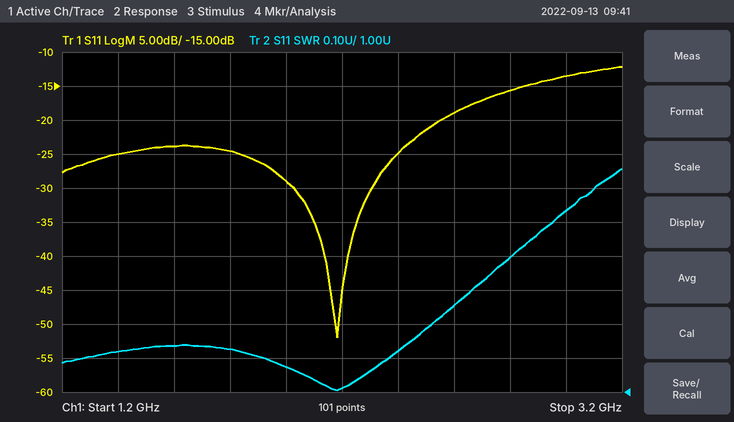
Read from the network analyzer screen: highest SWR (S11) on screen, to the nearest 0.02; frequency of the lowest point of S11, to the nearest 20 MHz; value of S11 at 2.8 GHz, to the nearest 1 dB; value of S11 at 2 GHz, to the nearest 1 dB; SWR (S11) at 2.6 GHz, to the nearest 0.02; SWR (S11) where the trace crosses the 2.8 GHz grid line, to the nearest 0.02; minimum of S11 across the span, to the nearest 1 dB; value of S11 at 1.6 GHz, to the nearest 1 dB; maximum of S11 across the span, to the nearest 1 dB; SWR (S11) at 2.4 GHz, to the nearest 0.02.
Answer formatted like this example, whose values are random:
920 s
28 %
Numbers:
1.66
2.18 GHz
-16 dB
-29 dB
1.26
1.40
-52 dB
-24 dB
-12 dB
1.12
